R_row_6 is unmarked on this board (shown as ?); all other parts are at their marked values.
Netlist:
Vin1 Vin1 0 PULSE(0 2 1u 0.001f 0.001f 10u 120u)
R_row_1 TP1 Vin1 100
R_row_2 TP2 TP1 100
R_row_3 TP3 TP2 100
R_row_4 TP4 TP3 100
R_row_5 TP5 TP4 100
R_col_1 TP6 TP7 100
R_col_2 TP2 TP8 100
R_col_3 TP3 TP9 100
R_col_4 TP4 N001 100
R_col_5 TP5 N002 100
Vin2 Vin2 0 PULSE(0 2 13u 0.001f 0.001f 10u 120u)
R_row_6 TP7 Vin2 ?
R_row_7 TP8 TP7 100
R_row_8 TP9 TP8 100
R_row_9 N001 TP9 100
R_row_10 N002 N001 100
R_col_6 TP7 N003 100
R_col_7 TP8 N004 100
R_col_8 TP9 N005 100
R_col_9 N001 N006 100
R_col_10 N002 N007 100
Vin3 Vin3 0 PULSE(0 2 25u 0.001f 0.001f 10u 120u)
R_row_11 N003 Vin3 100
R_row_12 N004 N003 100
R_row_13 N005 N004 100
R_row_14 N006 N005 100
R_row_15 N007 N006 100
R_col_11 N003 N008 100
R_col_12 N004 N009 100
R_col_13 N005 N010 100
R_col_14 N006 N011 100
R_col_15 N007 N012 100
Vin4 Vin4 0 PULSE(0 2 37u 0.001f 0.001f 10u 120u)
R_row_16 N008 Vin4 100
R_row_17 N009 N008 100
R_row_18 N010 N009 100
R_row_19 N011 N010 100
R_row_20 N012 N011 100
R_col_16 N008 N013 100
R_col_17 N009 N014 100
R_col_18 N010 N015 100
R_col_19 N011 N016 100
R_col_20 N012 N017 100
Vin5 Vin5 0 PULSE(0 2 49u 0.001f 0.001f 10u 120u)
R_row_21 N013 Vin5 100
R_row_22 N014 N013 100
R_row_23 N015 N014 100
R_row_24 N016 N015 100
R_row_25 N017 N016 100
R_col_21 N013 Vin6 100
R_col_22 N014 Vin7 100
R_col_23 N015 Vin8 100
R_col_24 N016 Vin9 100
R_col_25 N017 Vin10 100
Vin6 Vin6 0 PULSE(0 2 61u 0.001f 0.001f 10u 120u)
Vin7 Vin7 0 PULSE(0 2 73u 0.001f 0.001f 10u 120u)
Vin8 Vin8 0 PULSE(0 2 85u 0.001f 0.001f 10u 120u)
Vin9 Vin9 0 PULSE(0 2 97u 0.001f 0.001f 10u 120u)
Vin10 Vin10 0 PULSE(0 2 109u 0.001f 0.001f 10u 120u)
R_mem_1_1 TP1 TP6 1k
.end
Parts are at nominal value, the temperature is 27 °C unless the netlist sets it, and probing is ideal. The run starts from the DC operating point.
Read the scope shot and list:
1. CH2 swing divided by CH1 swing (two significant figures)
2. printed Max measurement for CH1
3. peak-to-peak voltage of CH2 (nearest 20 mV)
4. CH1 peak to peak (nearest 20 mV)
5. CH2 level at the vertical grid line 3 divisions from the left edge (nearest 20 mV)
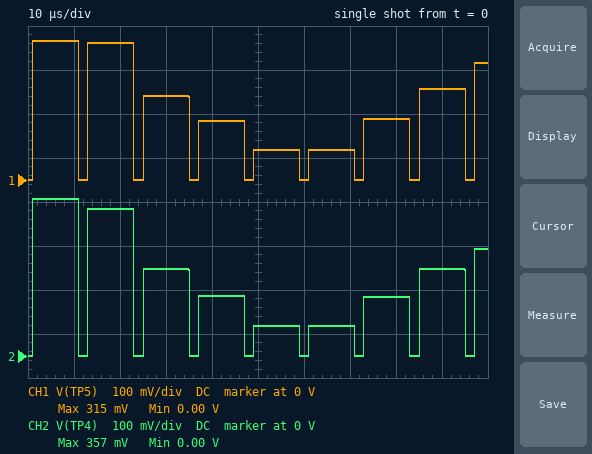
1.1
315 mV
360 mV
320 mV
200 mV
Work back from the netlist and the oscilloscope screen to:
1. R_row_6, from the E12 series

68 Ω
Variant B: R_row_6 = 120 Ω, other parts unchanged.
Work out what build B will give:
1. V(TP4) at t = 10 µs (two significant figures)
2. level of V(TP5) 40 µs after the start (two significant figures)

370 mV
140 mV
